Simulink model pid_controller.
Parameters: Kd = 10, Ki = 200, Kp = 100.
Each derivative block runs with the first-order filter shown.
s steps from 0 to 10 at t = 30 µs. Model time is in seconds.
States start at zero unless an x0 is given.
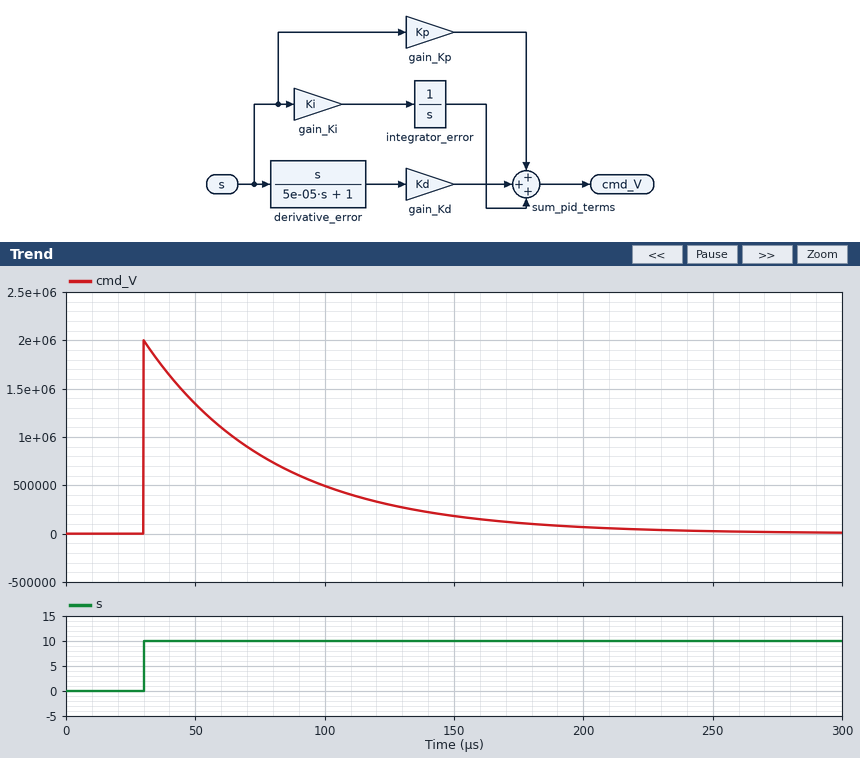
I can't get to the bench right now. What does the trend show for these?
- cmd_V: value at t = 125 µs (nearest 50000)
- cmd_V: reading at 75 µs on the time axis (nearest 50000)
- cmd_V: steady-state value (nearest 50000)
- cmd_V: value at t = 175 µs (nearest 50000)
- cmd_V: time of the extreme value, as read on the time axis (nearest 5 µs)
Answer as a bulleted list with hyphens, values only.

- 300000
- 800000
- 0
- 100000
- 30 µs
